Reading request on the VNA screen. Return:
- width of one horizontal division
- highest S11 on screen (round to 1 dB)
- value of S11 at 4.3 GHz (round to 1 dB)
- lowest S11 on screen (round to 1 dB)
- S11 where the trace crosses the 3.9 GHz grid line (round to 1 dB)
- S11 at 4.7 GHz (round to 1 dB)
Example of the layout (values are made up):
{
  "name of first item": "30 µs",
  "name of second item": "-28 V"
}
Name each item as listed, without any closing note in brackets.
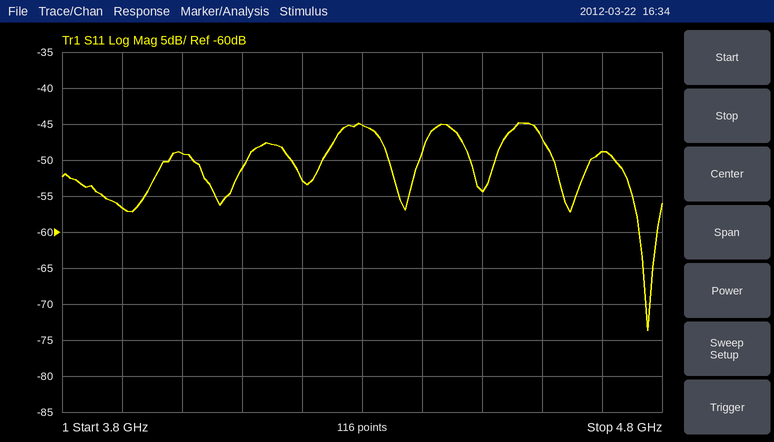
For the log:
{
  "width of one horizontal division": "100 MHz",
  "highest S11 on screen": "-45 dB",
  "value of S11 at 4.3 GHz": "-45 dB",
  "lowest S11 on screen": "-74 dB",
  "S11 where the trace crosses the 3.9 GHz grid line": "-57 dB",
  "S11 at 4.7 GHz": "-49 dB"
}
